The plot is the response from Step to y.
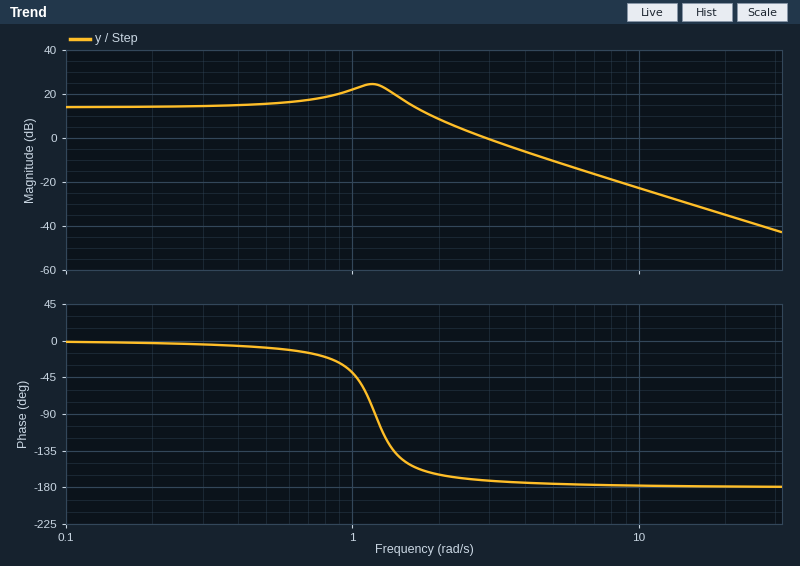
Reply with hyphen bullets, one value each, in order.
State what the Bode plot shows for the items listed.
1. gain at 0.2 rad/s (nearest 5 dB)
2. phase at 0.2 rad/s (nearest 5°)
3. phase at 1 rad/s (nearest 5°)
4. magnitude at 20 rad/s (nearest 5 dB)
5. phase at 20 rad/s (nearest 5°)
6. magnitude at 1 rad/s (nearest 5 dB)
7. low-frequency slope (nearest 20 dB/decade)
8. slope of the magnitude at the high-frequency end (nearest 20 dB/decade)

- 15 dB
- -5°
- -40°
- -35 dB
- -180°
- 20 dB
- 0 dB/decade
- -40 dB/decade
